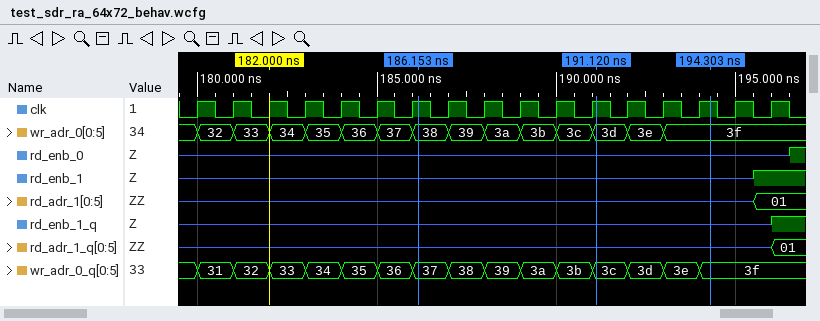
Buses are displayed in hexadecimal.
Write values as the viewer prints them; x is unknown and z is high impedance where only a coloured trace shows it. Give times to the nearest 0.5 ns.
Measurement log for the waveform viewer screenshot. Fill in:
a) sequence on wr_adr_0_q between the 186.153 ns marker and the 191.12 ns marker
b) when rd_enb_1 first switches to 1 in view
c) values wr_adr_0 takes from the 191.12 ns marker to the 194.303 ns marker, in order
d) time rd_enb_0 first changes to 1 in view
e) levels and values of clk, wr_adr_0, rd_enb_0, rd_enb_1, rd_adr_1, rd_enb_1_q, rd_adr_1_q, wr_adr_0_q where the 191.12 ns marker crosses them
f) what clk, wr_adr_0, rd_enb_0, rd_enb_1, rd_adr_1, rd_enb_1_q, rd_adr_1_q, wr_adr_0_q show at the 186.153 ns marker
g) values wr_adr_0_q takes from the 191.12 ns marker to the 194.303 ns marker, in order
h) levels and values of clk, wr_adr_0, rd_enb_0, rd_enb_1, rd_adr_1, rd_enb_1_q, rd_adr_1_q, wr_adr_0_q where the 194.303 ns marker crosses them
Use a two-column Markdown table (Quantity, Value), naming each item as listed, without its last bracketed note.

| Quantity | Value |
|---|---|
| sequence on wr_adr_0_q between the 186.153 ns marker and the 191.12 ns marker | 37, 38, 39, 3a, 3b, 3c |
| when rd_enb_1 first switches to 1 in view | 195.5 ns |
| values wr_adr_0 takes from the 191.12 ns marker to the 194.303 ns marker, in order | 3d, 3e, 3f |
| time rd_enb_0 first changes to 1 in view | 196.5 ns |
| levels and values of clk, wr_adr_0, rd_enb_0, rd_enb_1, rd_adr_1, rd_enb_1_q, rd_adr_1_q, wr_adr_0_q where the 191.12 ns marker crosses them | clk=1, wr_adr_0=3d, rd_enb_0=z, rd_enb_1=z, rd_adr_1=z, rd_enb_1_q=z, rd_adr_1_q=z, wr_adr_0_q=3c |
| what clk, wr_adr_0, rd_enb_0, rd_enb_1, rd_adr_1, rd_enb_1_q, rd_adr_1_q, wr_adr_0_q show at the 186.153 ns marker | clk=1, wr_adr_0=38, rd_enb_0=z, rd_enb_1=z, rd_adr_1=z, rd_enb_1_q=z, rd_adr_1_q=z, wr_adr_0_q=37 |
| values wr_adr_0_q takes from the 191.12 ns marker to the 194.303 ns marker, in order | 3c, 3d, 3e, 3f |
| levels and values of clk, wr_adr_0, rd_enb_0, rd_enb_1, rd_adr_1, rd_enb_1_q, rd_adr_1_q, wr_adr_0_q where the 194.303 ns marker crosses them | clk=1, wr_adr_0=3f, rd_enb_0=z, rd_enb_1=z, rd_adr_1=z, rd_enb_1_q=z, rd_adr_1_q=z, wr_adr_0_q=3f |
